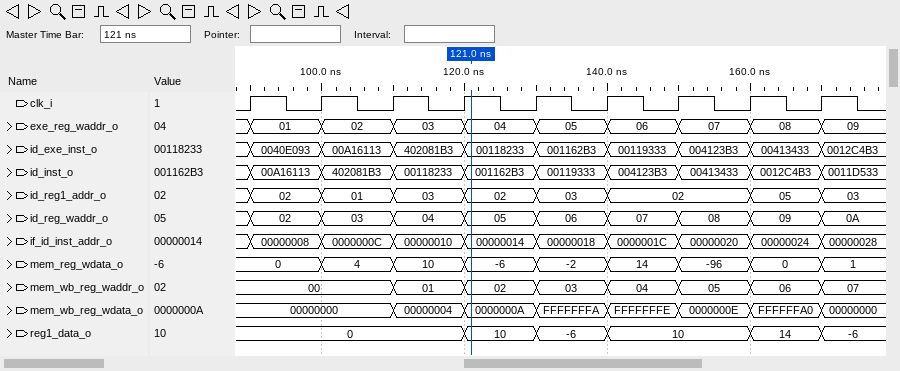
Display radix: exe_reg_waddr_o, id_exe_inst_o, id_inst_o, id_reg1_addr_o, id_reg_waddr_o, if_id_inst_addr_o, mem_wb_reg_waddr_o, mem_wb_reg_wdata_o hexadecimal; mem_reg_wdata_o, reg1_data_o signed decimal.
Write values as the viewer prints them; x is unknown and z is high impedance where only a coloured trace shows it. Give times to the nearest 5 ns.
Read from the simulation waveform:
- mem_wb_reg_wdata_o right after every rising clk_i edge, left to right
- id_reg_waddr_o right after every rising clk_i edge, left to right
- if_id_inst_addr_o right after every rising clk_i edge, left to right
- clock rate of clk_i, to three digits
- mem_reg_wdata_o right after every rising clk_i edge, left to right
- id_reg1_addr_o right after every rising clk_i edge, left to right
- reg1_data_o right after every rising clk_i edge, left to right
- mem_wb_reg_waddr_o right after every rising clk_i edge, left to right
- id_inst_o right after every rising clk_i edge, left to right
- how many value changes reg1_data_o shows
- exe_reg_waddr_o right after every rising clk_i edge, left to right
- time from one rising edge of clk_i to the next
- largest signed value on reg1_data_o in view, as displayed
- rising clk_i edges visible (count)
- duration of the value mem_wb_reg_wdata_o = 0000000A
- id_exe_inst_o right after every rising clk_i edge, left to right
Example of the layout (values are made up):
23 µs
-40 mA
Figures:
00000000, 00000000, 00000004, 0000000A, FFFFFFFA, FFFFFFFE, 0000000E, FFFFFFA0, 00000000
02, 03, 04, 05, 06, 07, 08, 09, 0A
00000008, 0000000C, 00000010, 00000014, 00000018, 0000001C, 00000020, 00000024, 00000028
100 MHz
0, 4, 10, -6, -2, 14, -96, 0, 1
02, 01, 03, 02, 03, 02, 02, 05, 03
0, 0, 0, 10, -6, 10, 10, 14, -6
00, 00, 01, 02, 03, 04, 05, 06, 07
00A16113, 402081B3, 00118233, 001162B3, 00119333, 004123B3, 00413433, 0012C4B3, 0011D533
5
01, 02, 03, 04, 05, 06, 07, 08, 09
10 ns
14
9
10 ns
0040E093, 00A16113, 402081B3, 00118233, 001162B3, 00119333, 004123B3, 00413433, 0012C4B3
